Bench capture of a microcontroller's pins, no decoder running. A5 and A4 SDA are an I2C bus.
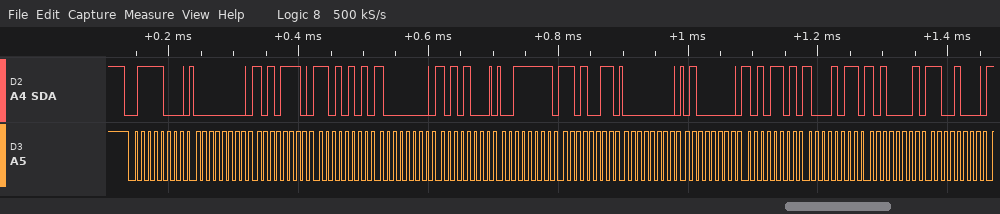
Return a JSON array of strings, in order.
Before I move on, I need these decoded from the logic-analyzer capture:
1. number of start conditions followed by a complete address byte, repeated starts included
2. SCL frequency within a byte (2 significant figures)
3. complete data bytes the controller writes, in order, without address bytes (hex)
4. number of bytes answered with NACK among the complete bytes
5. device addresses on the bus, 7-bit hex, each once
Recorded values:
["1", "100 kHz", "00 AE D5 80 A8 3F D3 00 40 AD 8B A1 C8", "0", "0x3C"]
